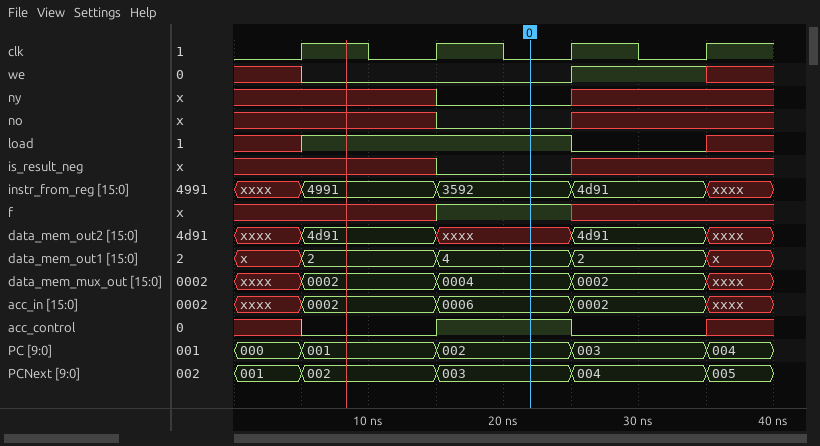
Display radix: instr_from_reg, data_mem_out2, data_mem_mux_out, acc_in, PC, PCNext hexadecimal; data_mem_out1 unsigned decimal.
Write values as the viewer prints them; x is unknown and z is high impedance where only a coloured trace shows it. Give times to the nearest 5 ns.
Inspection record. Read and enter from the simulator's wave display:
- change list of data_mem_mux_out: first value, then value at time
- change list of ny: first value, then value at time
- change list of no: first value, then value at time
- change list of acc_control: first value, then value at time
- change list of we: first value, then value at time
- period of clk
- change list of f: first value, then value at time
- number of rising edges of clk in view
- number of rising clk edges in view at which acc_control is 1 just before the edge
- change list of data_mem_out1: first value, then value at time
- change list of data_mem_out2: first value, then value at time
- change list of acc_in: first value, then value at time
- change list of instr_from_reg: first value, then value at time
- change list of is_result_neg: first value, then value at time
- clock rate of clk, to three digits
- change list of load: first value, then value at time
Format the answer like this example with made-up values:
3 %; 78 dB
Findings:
xxxx, 0002 at 5 ns, 0004 at 15 ns, 0002 at 25 ns, xxxx at 35 ns; x, 0 at 15 ns, x at 25 ns; x, 0 at 15 ns, x at 25 ns; x, 0 at 5 ns, 1 at 15 ns, 0 at 25 ns, x at 35 ns; x, 0 at 5 ns, 1 at 25 ns, x at 35 ns; 10 ns; x, 1 at 15 ns, x at 25 ns; 4; 1; x, 2 at 5 ns, 4 at 15 ns, 2 at 25 ns, x at 35 ns; xxxx, 4d91 at 5 ns, xxxx at 15 ns, 4d91 at 25 ns, xxxx at 35 ns; xxxx, 0002 at 5 ns, 0006 at 15 ns, 0002 at 25 ns, xxxx at 35 ns; xxxx, 4991 at 5 ns, 3592 at 15 ns, 4d91 at 25 ns, xxxx at 35 ns; x, 0 at 15 ns, x at 25 ns; 100 MHz; x, 1 at 5 ns, 0 at 25 ns, x at 35 ns
